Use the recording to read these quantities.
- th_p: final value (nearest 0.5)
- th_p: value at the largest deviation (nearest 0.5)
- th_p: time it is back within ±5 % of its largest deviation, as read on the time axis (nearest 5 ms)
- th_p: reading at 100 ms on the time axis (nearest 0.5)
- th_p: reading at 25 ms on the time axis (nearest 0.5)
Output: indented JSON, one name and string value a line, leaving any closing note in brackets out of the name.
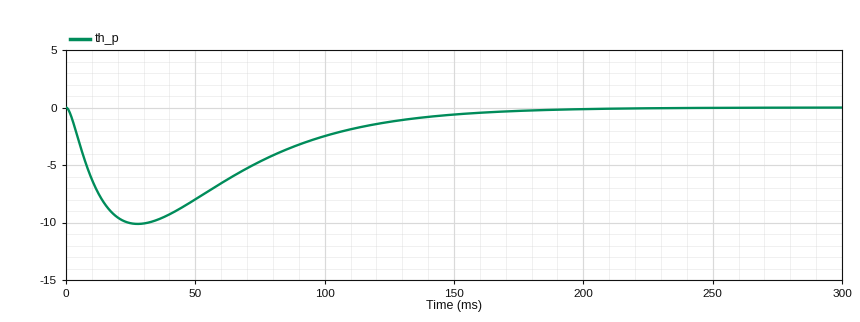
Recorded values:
{
  "th_p: final value": "0.0",
  "th_p: value at the largest deviation": "-10.0",
  "th_p: time it is back within ±5 % of its largest deviation, as read on the time axis": "155 ms",
  "th_p: reading at 100 ms on the time axis": "-2.5",
  "th_p: reading at 25 ms on the time axis": "-10.0"
}
